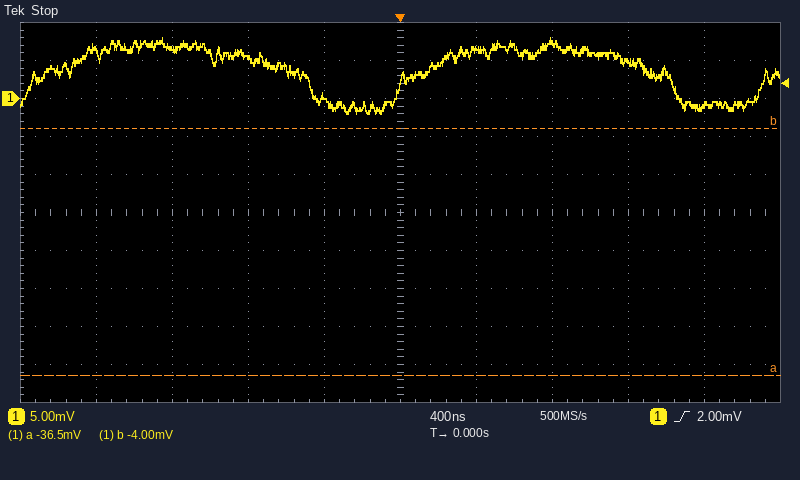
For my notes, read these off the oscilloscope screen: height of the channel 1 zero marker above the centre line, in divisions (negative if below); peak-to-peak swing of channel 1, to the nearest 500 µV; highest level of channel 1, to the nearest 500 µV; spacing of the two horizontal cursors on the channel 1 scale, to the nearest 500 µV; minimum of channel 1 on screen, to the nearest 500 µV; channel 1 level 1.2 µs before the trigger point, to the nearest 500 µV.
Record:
+3.0 div
10.0 mV
8.0 mV
32.5 mV
-2.0 mV
6.5 mV
